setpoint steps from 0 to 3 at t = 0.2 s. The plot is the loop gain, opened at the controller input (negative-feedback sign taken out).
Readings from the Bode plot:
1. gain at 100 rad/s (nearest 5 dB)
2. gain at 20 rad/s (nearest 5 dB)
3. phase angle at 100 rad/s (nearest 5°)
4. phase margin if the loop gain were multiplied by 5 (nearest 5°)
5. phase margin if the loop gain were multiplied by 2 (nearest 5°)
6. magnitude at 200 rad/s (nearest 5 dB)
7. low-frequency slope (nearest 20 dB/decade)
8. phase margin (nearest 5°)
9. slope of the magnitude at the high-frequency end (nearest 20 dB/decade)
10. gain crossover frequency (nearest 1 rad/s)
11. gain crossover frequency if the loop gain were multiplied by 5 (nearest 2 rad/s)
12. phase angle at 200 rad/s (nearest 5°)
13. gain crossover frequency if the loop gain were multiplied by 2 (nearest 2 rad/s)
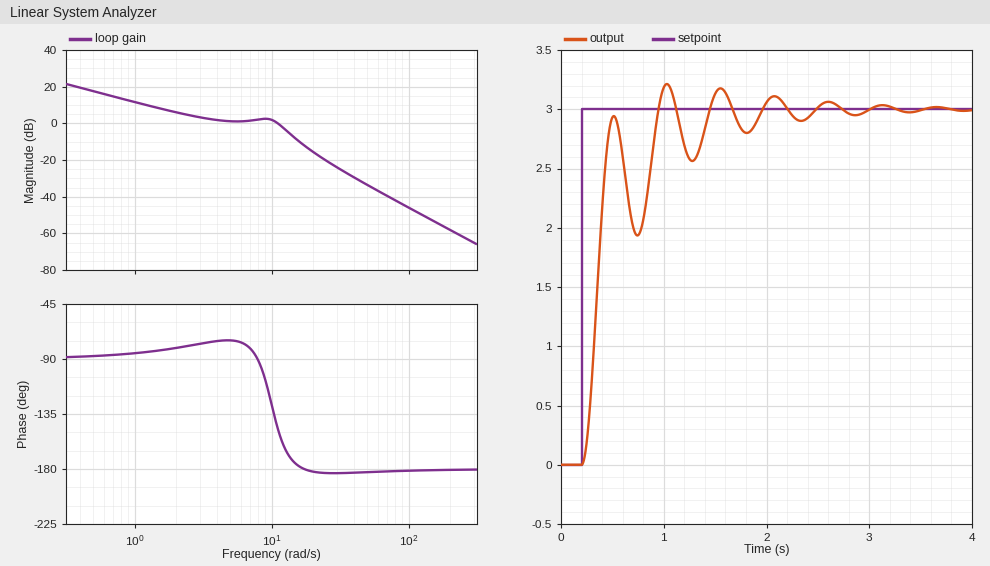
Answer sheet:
-45 dB
-15 dB
-180°
0°
10°
-60 dB
-20 dB/decade
35°
-40 dB/decade
11 rad/s
18 rad/s
-180°
14 rad/s
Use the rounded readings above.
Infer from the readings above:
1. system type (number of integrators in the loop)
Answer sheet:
1
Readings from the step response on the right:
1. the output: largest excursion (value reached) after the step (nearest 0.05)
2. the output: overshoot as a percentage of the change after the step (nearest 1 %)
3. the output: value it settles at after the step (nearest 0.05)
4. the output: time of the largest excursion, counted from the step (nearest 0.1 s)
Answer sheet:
3.20
7 %
3.00
0.8 s
